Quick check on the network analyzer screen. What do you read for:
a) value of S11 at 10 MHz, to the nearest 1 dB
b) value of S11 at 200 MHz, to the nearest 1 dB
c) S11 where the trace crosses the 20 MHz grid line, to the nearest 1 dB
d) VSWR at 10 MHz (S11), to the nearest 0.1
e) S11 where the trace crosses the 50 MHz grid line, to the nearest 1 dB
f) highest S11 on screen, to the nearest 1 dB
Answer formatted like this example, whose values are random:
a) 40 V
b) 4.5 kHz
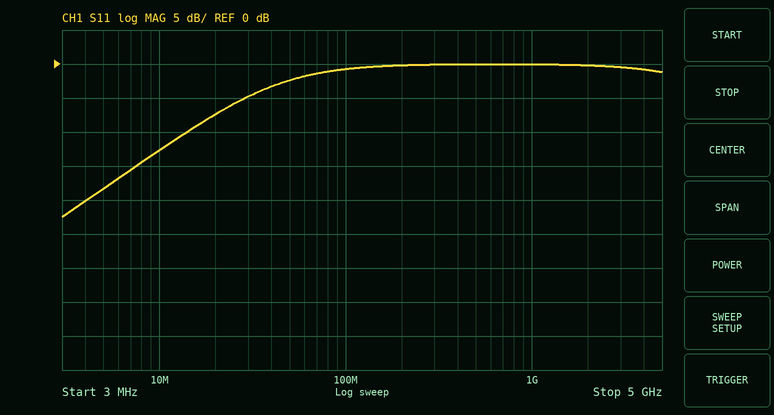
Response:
a) -13 dB
b) 0 dB
c) -7 dB
d) 1.6
e) -2 dB
f) 0 dB
